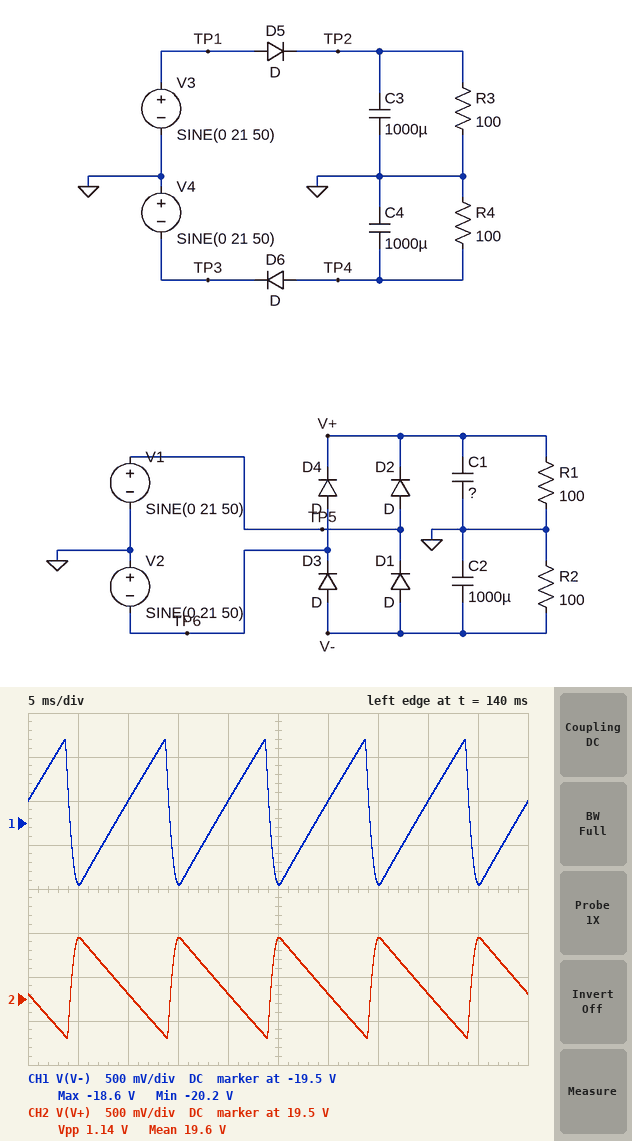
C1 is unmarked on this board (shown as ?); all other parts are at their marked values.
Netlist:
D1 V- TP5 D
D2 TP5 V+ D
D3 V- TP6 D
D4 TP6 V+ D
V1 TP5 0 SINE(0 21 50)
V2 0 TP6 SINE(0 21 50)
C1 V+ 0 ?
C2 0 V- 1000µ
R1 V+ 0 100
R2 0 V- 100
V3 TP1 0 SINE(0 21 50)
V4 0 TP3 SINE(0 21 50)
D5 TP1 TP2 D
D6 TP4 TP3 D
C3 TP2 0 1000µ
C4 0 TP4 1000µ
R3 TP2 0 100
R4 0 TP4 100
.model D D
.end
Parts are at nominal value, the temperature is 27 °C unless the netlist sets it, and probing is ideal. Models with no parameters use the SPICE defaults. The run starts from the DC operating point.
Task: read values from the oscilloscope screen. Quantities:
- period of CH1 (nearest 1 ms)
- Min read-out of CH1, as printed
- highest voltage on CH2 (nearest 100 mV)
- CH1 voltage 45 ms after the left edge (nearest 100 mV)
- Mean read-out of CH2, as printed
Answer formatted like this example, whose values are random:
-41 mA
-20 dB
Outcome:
10 ms
-20.2 V
20.2 V
-20.2 V
19.6 V
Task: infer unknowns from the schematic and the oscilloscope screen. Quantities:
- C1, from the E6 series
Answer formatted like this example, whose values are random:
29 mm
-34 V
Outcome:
1.5 mF
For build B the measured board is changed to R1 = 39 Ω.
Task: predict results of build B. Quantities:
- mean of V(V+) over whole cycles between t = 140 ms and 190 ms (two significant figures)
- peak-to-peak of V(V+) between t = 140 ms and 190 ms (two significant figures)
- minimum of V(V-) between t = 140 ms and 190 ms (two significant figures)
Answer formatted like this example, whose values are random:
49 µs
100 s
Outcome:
19 V
2.6 V
-20 V
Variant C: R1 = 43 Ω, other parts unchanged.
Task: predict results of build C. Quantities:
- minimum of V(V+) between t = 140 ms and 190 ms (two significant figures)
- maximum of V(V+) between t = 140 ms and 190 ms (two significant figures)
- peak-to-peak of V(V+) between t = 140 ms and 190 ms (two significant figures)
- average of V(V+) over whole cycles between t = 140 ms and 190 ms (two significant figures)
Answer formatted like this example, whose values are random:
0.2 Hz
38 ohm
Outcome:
18 V
20 V
2.4 V
19 V
